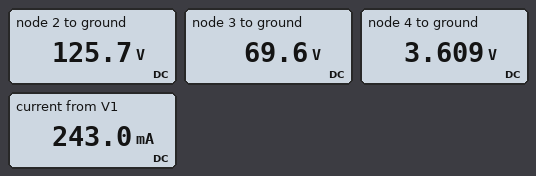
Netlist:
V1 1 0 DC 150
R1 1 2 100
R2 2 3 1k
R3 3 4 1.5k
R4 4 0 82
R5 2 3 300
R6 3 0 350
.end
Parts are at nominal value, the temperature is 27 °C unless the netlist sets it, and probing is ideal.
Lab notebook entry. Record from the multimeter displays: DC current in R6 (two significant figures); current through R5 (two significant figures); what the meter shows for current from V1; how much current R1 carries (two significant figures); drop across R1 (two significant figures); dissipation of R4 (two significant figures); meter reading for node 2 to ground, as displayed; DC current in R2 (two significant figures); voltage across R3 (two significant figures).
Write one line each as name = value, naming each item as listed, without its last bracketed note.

DC current in R6 = 200 mA
current through R5 = 190 mA
what the meter shows for current from V1 = 243.0 mA
how much current R1 carries = 240 mA
drop across R1 = 24 V
dissipation of R4 = 160 mW
meter reading for node 2 to ground, as displayed = 125.7 V
DC current in R2 = 56 mA
voltage across R3 = 66 V
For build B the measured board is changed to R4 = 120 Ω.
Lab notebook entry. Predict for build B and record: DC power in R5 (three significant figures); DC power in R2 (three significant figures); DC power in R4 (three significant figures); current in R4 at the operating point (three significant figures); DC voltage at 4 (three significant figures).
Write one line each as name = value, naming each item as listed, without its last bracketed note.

DC power in R5 = 10.4 W
DC power in R2 = 3.13 W
DC power in R4 = 223 mW
current in R4 at the operating point = 43.1 mA
DC voltage at 4 = 5.17 V
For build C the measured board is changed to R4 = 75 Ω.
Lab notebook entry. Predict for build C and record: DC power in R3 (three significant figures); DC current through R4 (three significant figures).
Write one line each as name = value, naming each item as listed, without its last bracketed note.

DC power in R3 = 2.93 W
DC current through R4 = 44.2 mA
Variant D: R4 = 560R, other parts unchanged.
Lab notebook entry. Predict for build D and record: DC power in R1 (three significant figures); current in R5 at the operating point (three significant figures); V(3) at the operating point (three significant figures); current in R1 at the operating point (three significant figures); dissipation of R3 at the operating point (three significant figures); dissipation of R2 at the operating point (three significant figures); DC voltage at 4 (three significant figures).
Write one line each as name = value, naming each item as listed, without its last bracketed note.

DC power in R1 = 5.67 W
current in R5 at the operating point = 183 mA
V(3) at the operating point = 71.2 V
current in R1 at the operating point = 238 mA
dissipation of R3 at the operating point = 1.79 W
dissipation of R2 at the operating point = 3.02 W
DC voltage at 4 = 19.4 V
